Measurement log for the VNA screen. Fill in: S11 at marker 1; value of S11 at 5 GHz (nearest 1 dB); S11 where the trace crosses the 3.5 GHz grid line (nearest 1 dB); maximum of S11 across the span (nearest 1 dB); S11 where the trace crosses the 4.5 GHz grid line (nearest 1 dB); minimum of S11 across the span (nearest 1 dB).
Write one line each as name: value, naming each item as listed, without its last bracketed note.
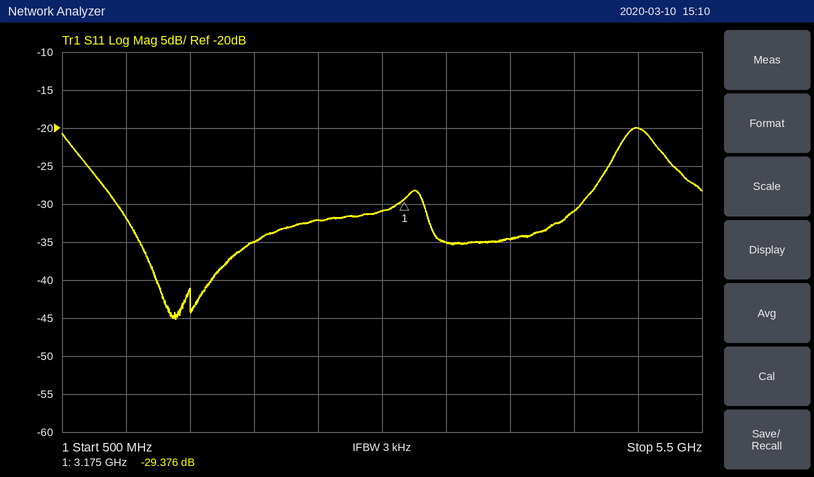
S11 at marker 1: -29.376 dB
value of S11 at 5 GHz: -20 dB
S11 where the trace crosses the 3.5 GHz grid line: -35 dB
maximum of S11 across the span: -20 dB
S11 where the trace crosses the 4.5 GHz grid line: -31 dB
minimum of S11 across the span: -45 dB
